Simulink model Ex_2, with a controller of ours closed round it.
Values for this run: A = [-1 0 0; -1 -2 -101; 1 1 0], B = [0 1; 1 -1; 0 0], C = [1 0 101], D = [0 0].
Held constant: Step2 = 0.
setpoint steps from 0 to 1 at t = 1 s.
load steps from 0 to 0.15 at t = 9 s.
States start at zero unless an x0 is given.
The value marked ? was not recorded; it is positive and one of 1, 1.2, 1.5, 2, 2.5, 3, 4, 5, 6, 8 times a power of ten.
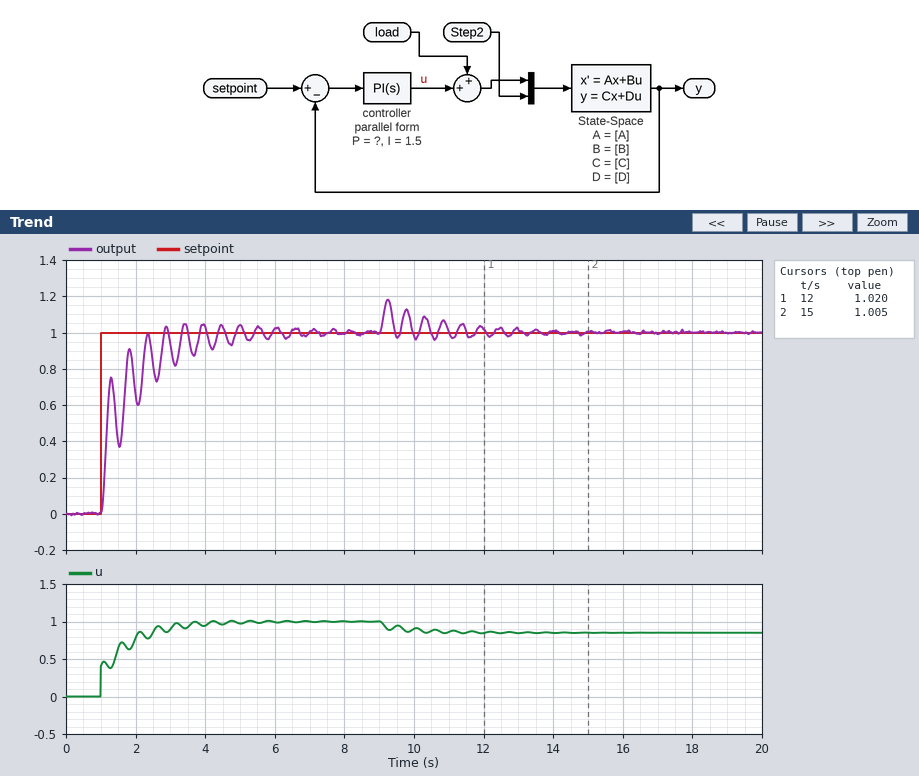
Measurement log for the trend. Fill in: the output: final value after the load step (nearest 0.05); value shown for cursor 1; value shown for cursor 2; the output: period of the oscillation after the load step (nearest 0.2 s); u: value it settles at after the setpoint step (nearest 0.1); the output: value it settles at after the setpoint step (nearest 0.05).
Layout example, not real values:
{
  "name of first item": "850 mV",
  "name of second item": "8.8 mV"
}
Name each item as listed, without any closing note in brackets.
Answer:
{
  "the output: final value after the load step": "1.00",
  "value shown for cursor 1": "1.020",
  "value shown for cursor 2": "1.005",
  "the output: period of the oscillation after the load step": "0.6 s",
  "u: value it settles at after the setpoint step": "1.0",
  "the output: value it settles at after the setpoint step": "1.00"
}
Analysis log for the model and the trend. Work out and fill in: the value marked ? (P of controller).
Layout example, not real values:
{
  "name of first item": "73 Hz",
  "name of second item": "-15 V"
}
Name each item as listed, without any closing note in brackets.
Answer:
{
  "the value marked ?": "0.4"
}
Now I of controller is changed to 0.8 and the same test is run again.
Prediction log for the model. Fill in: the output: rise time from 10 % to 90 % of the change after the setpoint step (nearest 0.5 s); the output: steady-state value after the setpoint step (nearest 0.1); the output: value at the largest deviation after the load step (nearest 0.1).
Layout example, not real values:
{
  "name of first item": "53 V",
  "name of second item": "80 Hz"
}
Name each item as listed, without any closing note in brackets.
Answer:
{
  "the output: rise time from 10 % to 90 % of the change after the setpoint step": "3.0 s",
  "the output: steady-state value after the setpoint step": "1.0",
  "the output: value at the largest deviation after the load step": "1.2"
}
